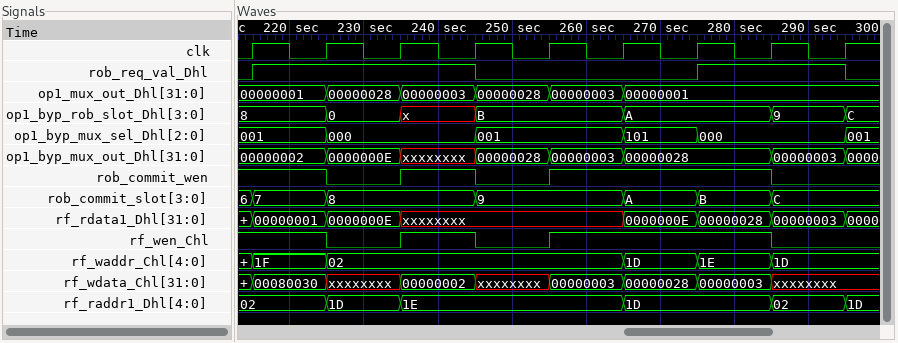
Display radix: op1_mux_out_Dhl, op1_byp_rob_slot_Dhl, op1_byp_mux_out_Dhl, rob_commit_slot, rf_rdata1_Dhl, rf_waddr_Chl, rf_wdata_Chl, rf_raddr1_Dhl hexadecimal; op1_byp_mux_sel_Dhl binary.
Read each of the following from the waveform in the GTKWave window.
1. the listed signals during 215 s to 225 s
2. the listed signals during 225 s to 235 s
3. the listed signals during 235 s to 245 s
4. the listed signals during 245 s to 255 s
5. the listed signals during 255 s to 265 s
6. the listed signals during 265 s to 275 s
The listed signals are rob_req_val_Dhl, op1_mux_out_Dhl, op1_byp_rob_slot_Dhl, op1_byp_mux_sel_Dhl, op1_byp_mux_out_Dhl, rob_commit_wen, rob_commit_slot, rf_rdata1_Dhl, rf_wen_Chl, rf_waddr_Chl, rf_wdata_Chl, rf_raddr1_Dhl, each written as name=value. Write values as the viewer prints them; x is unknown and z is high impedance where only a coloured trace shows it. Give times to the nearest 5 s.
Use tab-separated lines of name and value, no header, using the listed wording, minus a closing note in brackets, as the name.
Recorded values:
the listed signals during 215 s to 225 s	rob_req_val_Dhl=1, op1_mux_out_Dhl=00000001, op1_byp_rob_slot_Dhl=8, op1_byp_mux_sel_Dhl=001, op1_byp_mux_out_Dhl=00000002, rob_commit_wen=1, rob_commit_slot=7, rf_rdata1_Dhl=00000001, rf_wen_Chl=1, rf_waddr_Chl=1F, rf_wdata_Chl=00080030, rf_raddr1_Dhl=02
the listed signals during 225 s to 235 s	rob_req_val_Dhl=1, op1_mux_out_Dhl=00000028, op1_byp_rob_slot_Dhl=0, op1_byp_mux_sel_Dhl=000, op1_byp_mux_out_Dhl=0000000E, rob_commit_wen=0, rob_commit_slot=8, rf_rdata1_Dhl=0000000E, rf_wen_Chl=0, rf_waddr_Chl=02, rf_wdata_Chl=xxxxxxxx, rf_raddr1_Dhl=1D
the listed signals during 235 s to 245 s	rob_req_val_Dhl=1, op1_mux_out_Dhl=00000003, op1_byp_rob_slot_Dhl=x, op1_byp_mux_sel_Dhl=000, op1_byp_mux_out_Dhl=xxxxxxxx, rob_commit_wen=1, rob_commit_slot=8, rf_rdata1_Dhl=xxxxxxxx, rf_wen_Chl=1, rf_waddr_Chl=02, rf_wdata_Chl=00000002, rf_raddr1_Dhl=1E
the listed signals during 245 s to 255 s	rob_req_val_Dhl=0, op1_mux_out_Dhl=00000028, op1_byp_rob_slot_Dhl=B, op1_byp_mux_sel_Dhl=001, op1_byp_mux_out_Dhl=00000028, rob_commit_wen=0, rob_commit_slot=9, rf_rdata1_Dhl=xxxxxxxx, rf_wen_Chl=0, rf_waddr_Chl=02, rf_wdata_Chl=xxxxxxxx, rf_raddr1_Dhl=1E
the listed signals during 255 s to 265 s	rob_req_val_Dhl=0, op1_mux_out_Dhl=00000003, op1_byp_rob_slot_Dhl=B, op1_byp_mux_sel_Dhl=001, op1_byp_mux_out_Dhl=00000003, rob_commit_wen=1, rob_commit_slot=9, rf_rdata1_Dhl=xxxxxxxx, rf_wen_Chl=1, rf_waddr_Chl=02, rf_wdata_Chl=00000003, rf_raddr1_Dhl=1E
the listed signals during 265 s to 275 s	rob_req_val_Dhl=0, op1_mux_out_Dhl=00000001, op1_byp_rob_slot_Dhl=A, op1_byp_mux_sel_Dhl=101, op1_byp_mux_out_Dhl=00000028, rob_commit_wen=1, rob_commit_slot=A, rf_rdata1_Dhl=0000000E, rf_wen_Chl=1, rf_waddr_Chl=1D, rf_wdata_Chl=00000028, rf_raddr1_Dhl=1D
